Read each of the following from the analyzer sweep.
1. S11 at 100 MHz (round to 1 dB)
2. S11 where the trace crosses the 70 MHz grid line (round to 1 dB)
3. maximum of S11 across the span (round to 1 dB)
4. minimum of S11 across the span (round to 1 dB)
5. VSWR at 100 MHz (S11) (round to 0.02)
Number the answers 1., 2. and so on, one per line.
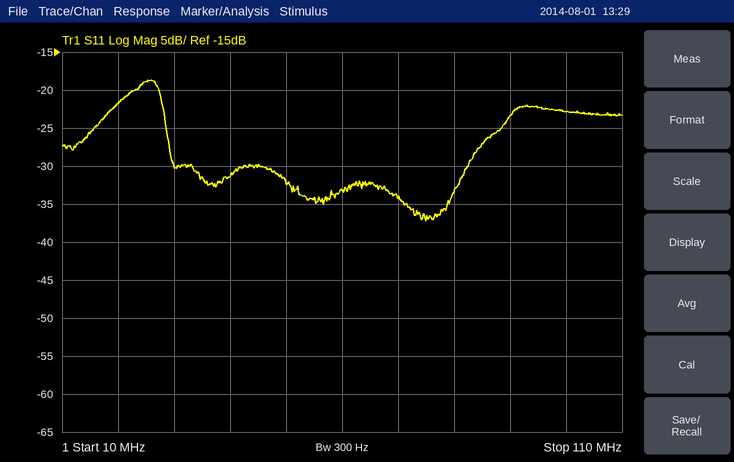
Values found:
1. -23 dB
2. -34 dB
3. -19 dB
4. -37 dB
5. 1.16
